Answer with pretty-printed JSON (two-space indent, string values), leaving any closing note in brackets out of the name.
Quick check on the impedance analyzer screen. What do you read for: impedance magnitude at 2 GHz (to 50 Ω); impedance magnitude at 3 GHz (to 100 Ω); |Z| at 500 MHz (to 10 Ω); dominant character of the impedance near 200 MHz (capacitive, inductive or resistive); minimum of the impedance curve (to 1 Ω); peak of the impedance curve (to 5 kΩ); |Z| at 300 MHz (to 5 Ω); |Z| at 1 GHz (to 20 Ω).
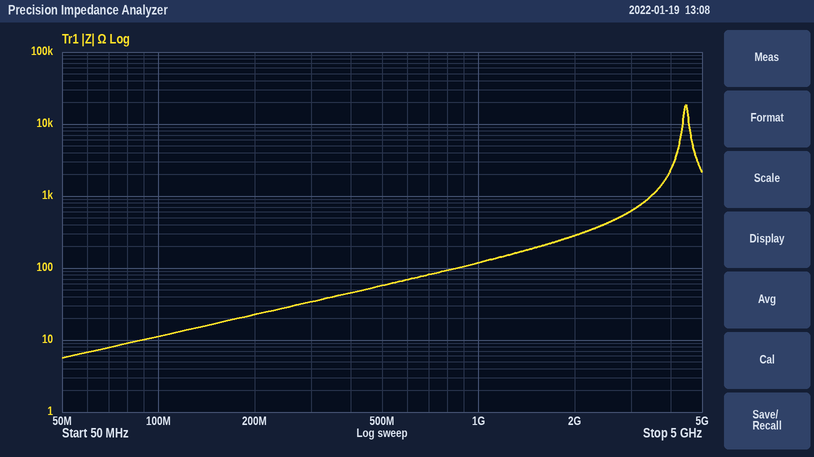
{
  "impedance magnitude at 2 GHz": "300 Ω",
  "impedance magnitude at 3 GHz": "600 Ω",
  "|Z| at 500 MHz": "60 Ω",
  "dominant character of the impedance near 200 MHz": "inductive",
  "minimum of the impedance curve": "6 Ω",
  "peak of the impedance curve": "20 kΩ",
  "|Z| at 300 MHz": "35 Ω",
  "|Z| at 1 GHz": "120 Ω"
}
